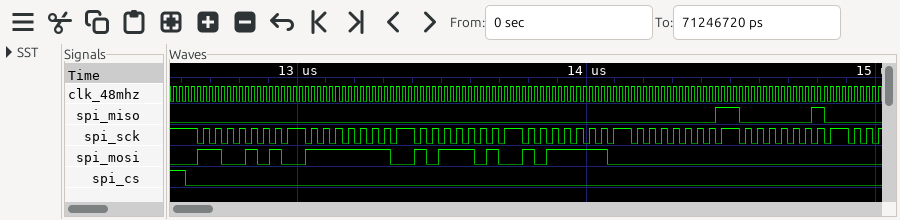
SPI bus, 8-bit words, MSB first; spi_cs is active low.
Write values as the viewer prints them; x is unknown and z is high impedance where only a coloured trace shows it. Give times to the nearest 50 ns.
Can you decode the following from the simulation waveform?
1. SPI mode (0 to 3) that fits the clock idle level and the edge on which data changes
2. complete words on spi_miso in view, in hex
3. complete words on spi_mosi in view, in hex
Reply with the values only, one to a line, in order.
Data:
3
00, 00, 00, 00, 01, 02
CA, FE, BA, BE, 00, 00
